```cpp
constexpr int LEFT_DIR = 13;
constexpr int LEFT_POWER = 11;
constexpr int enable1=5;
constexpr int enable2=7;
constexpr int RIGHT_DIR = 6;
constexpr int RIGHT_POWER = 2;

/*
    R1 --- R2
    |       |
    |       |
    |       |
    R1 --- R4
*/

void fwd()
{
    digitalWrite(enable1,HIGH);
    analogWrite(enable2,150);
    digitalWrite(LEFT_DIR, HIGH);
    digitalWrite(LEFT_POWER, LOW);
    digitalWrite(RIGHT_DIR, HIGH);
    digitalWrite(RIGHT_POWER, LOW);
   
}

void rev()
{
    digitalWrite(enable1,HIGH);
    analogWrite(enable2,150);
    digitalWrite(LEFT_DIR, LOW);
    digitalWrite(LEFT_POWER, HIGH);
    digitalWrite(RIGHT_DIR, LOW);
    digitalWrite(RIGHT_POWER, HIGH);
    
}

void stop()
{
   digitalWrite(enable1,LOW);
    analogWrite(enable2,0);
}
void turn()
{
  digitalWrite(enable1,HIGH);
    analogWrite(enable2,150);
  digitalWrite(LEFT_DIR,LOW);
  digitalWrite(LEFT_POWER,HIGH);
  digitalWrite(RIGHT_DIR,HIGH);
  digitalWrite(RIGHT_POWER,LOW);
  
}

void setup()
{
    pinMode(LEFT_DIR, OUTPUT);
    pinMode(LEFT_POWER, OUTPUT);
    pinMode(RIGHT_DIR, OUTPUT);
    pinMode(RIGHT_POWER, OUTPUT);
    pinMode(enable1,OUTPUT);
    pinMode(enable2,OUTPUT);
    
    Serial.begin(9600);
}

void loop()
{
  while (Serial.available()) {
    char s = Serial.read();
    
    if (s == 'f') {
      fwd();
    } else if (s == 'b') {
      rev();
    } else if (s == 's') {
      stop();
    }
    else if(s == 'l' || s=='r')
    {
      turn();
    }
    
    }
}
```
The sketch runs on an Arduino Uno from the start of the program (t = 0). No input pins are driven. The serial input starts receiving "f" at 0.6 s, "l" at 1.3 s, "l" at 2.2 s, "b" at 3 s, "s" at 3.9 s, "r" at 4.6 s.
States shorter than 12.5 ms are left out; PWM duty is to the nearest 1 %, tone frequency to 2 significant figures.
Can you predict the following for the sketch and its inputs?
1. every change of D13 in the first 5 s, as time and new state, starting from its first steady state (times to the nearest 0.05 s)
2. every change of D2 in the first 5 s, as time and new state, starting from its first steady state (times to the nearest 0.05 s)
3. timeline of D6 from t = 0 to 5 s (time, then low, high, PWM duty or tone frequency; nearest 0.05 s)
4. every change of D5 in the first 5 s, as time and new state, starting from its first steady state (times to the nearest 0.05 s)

0 s low; 0.6 s high; 1.3 s low
0 s low; 3 s high; 4.6 s low
0 s low; 0.6 s high; 3 s low; 4.6 s high
0 s low; 0.6 s high; 3.9 s low; 4.6 s high
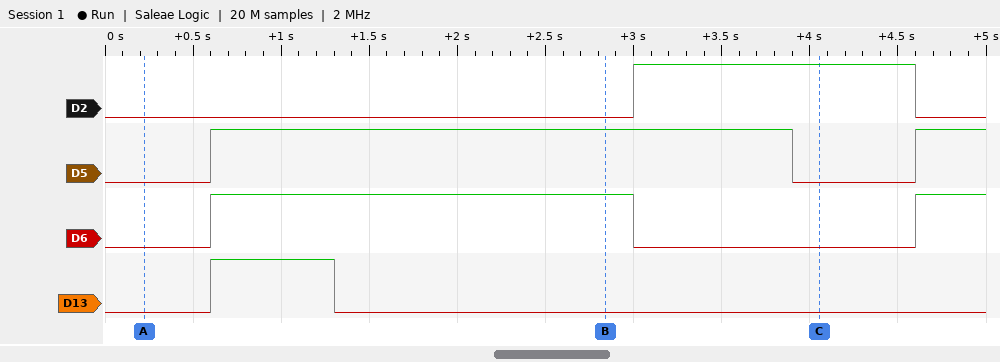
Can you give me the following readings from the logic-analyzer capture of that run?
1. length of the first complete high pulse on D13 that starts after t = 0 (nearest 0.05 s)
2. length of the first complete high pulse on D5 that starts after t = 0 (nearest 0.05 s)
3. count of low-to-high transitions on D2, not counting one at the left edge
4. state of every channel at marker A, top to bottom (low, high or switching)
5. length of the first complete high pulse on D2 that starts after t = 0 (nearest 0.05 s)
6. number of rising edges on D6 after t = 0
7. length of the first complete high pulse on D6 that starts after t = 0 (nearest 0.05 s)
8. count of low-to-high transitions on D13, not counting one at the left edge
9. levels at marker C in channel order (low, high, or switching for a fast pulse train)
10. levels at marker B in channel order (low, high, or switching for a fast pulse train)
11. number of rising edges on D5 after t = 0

0.70 s
3.30 s
1
D2 low, D5 low, D6 low, D13 low
1.60 s
2
2.40 s
1
D2 high, D5 low, D6 low, D13 low
D2 low, D5 high, D6 high, D13 low
2
